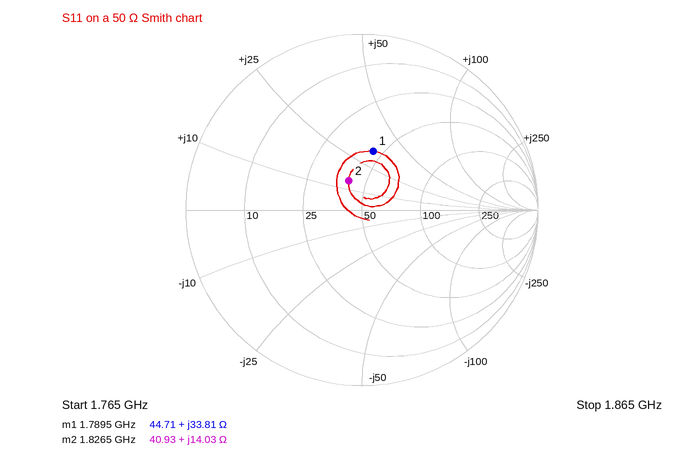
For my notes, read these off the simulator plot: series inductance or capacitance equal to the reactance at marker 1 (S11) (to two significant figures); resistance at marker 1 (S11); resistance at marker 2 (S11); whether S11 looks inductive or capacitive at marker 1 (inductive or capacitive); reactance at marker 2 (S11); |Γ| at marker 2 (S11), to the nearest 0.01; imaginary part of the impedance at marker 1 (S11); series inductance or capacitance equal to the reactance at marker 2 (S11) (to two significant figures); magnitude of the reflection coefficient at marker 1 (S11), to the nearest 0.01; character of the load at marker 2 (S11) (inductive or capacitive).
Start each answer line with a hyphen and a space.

- 3.0 nH
- 44.71 Ω
- 40.93 Ω
- inductive
- +14.03 Ω
- 0.18
- +33.81 Ω
- 1.2 nH
- 0.34
- inductive
